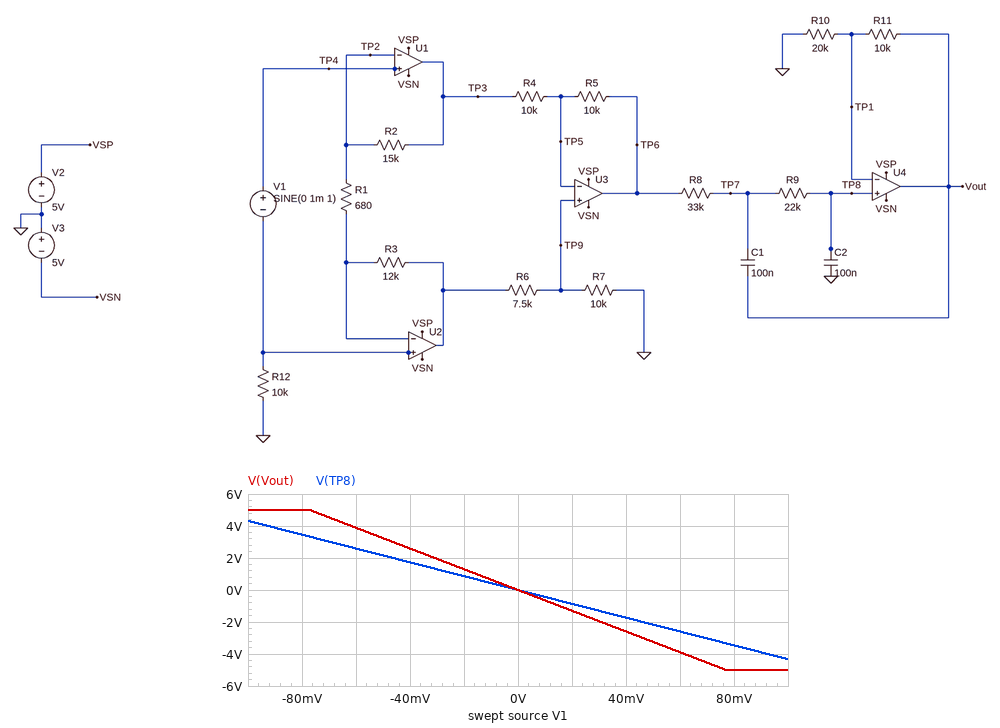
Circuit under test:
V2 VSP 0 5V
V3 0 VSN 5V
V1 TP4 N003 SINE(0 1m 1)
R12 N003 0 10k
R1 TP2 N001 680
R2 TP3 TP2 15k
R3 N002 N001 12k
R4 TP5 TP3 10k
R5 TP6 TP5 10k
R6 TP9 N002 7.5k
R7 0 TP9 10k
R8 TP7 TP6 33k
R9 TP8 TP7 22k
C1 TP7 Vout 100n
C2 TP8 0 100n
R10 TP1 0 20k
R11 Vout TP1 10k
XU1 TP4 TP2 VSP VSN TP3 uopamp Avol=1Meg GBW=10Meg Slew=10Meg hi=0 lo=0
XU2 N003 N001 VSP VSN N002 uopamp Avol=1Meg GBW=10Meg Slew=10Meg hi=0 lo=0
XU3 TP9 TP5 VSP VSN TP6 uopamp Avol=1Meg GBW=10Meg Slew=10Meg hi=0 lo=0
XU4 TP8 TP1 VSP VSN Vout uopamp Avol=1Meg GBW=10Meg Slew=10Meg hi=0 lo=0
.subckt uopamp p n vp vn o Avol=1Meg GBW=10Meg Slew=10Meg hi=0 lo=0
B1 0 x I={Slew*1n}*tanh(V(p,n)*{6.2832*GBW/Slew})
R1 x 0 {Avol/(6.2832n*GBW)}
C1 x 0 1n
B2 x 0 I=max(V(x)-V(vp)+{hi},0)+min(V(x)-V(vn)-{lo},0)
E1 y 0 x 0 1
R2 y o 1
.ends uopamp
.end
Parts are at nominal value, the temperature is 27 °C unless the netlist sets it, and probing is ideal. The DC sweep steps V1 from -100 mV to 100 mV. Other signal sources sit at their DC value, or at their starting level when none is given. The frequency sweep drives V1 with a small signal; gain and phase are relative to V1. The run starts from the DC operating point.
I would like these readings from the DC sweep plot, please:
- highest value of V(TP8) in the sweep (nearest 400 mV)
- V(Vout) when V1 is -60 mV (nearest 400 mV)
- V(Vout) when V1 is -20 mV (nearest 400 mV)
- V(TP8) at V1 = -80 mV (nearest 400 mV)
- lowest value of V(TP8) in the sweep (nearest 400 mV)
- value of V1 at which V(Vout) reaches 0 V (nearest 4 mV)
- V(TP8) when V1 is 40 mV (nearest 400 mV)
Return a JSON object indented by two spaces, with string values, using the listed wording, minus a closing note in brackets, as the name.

{
  "highest value of V(TP8) in the sweep": "4.4 V",
  "V(Vout) when V1 is -60 mV": "4.0 V",
  "V(Vout) when V1 is -20 mV": "1.2 V",
  "V(TP8) at V1 = -80 mV": "3.6 V",
  "lowest value of V(TP8) in the sweep": "-4.4 V",
  "value of V1 at which V(Vout) reaches 0 V": "0 V",
  "V(TP8) when V1 is 40 mV": "-1.6 V"
}
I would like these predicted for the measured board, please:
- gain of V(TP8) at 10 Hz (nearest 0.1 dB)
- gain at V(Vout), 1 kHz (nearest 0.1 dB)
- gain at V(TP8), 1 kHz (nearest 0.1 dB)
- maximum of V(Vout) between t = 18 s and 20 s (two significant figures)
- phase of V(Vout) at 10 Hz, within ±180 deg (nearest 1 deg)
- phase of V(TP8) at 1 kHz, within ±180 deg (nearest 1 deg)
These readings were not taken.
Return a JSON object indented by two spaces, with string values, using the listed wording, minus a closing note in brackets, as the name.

{
  "gain of V(TP8) at 10 Hz": "32.7 dB",
  "gain at V(Vout), 1 kHz": "-12.9 dB",
  "gain at V(TP8), 1 kHz": "-16.4 dB",
  "maximum of V(Vout) between t = 18 s and 20 s": "65 mV",
  "phase of V(Vout) at 10 Hz, within ±180 deg": "166 deg",
  "phase of V(TP8) at 1 kHz, within ±180 deg": "5 deg"
}
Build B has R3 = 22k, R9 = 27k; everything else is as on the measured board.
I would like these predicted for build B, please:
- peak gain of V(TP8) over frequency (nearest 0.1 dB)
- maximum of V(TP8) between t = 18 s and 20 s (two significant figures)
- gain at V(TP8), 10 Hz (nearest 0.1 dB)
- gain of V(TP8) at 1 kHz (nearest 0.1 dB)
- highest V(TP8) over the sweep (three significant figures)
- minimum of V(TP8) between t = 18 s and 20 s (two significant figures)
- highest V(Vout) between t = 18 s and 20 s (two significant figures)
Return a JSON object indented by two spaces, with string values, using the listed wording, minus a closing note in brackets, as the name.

{
  "peak gain of V(TP8) over frequency": "35.6 dB",
  "maximum of V(TP8) between t = 18 s and 20 s": "60 mV",
  "gain at V(TP8), 10 Hz": "35.5 dB",
  "gain of V(TP8) at 1 kHz": "-15.4 dB",
  "highest V(TP8) over the sweep": "5.01 V",
  "minimum of V(TP8) between t = 18 s and 20 s": "-60 mV",
  "highest V(Vout) between t = 18 s and 20 s": "90 mV"
}
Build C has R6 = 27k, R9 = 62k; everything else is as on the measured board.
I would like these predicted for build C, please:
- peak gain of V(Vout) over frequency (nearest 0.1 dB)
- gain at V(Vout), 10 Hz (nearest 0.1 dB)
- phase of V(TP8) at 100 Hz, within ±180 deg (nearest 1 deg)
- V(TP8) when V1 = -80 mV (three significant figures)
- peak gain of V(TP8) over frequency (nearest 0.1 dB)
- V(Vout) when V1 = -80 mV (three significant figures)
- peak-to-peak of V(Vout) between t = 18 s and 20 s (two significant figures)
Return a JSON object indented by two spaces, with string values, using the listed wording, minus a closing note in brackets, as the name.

{
  "peak gain of V(Vout) over frequency": "33.8 dB",
  "gain at V(Vout), 10 Hz": "33.4 dB",
  "phase of V(TP8) at 100 Hz, within ±180 deg": "35 deg",
  "V(TP8) when V1 = -80 mV": "2.61 V",
  "peak gain of V(TP8) over frequency": "30.3 dB",
  "V(Vout) when V1 = -80 mV": "3.91 V",
  "peak-to-peak of V(Vout) between t = 18 s and 20 s": "98 mV"
}
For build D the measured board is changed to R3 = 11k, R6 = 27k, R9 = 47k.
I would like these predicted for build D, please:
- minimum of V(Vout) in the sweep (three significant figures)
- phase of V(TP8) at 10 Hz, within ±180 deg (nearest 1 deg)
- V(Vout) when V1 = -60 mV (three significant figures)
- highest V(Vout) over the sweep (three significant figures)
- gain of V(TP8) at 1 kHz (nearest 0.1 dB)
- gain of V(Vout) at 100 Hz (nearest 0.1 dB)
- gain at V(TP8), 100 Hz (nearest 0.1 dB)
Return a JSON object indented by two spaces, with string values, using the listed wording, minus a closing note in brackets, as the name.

{
  "minimum of V(Vout) in the sweep": "-4.77 V",
  "phase of V(TP8) at 10 Hz, within ±180 deg": "157 deg",
  "V(Vout) when V1 = -60 mV": "2.86 V",
  "highest V(Vout) over the sweep": "4.77 V",
  "gain of V(TP8) at 1 kHz": "-25.7 dB",
  "gain of V(Vout) at 100 Hz": "17.3 dB",
  "gain at V(TP8), 100 Hz": "13.8 dB"
}
